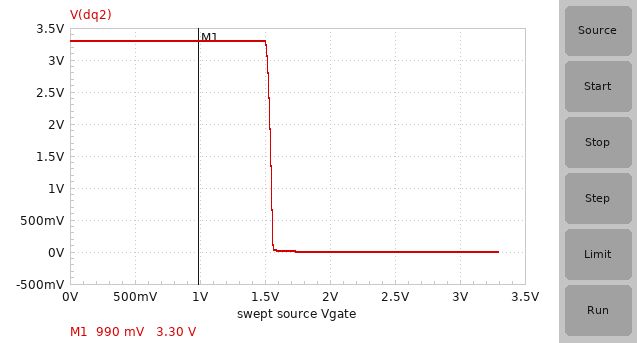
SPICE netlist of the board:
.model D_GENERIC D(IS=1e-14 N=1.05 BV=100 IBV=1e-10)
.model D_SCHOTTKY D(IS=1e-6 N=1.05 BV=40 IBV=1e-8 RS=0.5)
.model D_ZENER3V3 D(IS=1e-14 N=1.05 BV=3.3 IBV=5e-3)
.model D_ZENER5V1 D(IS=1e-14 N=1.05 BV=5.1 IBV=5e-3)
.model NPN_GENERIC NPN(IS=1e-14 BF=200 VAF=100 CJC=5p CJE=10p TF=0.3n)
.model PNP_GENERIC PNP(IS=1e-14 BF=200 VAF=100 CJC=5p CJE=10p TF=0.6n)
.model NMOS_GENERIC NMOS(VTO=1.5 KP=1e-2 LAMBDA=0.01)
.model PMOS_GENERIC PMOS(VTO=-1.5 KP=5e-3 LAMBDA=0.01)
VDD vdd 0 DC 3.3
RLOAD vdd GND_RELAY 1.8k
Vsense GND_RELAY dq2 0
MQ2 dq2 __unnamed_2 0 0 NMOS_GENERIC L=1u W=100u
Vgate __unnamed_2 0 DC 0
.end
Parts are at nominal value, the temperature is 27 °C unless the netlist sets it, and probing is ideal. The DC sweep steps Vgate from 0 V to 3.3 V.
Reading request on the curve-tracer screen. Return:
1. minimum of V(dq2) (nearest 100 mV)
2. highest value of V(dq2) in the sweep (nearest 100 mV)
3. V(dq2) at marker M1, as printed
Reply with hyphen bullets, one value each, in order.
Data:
- 0 V
- 3.3 V
- 3.30 V
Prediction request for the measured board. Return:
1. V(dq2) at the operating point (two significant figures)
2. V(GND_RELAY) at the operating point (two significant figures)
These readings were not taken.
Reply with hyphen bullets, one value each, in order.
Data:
- 3.3 V
- 3.3 V
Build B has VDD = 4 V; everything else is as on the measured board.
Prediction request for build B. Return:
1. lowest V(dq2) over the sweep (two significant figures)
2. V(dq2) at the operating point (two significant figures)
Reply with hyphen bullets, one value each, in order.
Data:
- 1.2 mV
- 4.0 V
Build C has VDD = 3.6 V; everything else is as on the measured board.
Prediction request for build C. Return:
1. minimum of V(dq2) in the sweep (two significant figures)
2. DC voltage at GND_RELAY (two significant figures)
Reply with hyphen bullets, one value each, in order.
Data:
- 1.1 mV
- 3.6 V
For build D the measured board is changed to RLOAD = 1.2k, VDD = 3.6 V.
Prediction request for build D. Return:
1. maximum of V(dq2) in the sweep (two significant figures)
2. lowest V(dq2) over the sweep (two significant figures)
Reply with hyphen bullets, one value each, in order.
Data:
- 3.6 V
- 1.7 mV
